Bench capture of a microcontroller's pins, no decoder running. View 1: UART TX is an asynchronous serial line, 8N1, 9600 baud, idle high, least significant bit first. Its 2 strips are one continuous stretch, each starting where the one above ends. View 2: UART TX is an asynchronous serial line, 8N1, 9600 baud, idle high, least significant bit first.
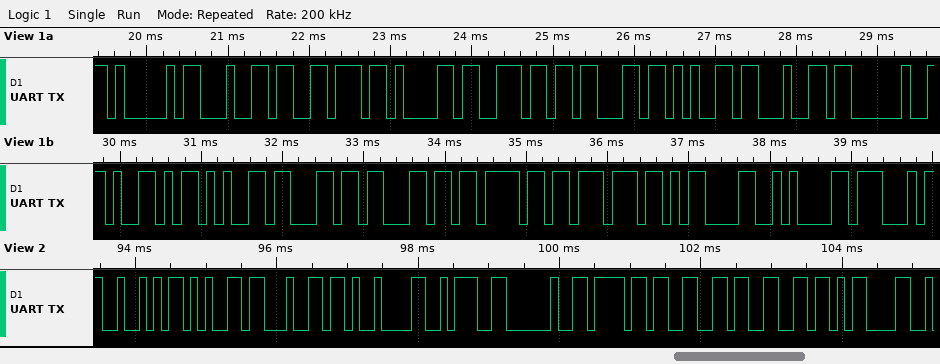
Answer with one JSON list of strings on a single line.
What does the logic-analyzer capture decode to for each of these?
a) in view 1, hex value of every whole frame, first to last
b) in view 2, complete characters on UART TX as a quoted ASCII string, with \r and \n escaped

["41 64 76 61 6E 63 65 64 20 59 65 6C 6C 6F 77 0D 0A 47", "\"Red\\t: off\\r\""]
